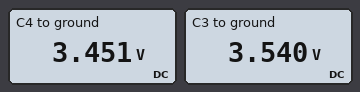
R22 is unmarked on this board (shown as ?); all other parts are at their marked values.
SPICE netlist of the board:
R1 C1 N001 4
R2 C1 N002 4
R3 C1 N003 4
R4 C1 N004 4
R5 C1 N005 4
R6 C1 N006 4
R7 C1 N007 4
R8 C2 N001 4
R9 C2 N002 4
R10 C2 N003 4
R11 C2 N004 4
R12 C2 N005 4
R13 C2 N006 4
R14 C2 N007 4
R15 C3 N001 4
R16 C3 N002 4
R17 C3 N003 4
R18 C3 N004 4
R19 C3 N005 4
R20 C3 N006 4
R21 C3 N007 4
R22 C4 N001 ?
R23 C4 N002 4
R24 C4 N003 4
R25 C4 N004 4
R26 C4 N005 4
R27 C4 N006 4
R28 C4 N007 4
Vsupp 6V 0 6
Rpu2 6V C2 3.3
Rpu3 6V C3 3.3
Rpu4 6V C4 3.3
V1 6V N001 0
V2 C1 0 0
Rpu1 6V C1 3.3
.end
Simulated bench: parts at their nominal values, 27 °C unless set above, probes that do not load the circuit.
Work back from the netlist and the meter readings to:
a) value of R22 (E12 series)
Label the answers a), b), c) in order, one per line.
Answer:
a) 5.6 Ω
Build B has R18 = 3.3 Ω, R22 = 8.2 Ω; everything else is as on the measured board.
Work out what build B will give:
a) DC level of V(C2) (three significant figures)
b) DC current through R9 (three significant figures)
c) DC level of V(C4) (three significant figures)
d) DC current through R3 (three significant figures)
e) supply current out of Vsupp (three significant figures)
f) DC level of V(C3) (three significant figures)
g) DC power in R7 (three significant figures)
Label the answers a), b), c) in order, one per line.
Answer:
a) 3.51 V
b) 231 mA
c) 3.35 V
d) 647 mA
e) 7.21 A
f) 3.49 V
g) 1.67 W
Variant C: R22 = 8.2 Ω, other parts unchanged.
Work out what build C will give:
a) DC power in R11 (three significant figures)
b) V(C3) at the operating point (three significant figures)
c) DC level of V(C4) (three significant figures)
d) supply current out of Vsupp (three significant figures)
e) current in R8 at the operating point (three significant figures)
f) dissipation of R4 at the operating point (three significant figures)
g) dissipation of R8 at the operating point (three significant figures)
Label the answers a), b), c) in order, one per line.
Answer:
a) 211 mW
b) 3.51 V
c) 3.34 V
d) 7.20 A
e) 623 mA
f) 1.68 W
g) 1.55 W
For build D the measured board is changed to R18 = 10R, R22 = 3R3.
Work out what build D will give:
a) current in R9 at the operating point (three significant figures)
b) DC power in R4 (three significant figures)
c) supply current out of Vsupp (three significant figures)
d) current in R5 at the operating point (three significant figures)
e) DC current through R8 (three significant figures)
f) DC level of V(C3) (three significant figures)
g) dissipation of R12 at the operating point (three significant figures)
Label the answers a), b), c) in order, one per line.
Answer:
a) 215 mA
b) 1.64 W
c) 7.37 A
d) 682 mA
e) 603 mA
f) 3.67 V
g) 186 mW
